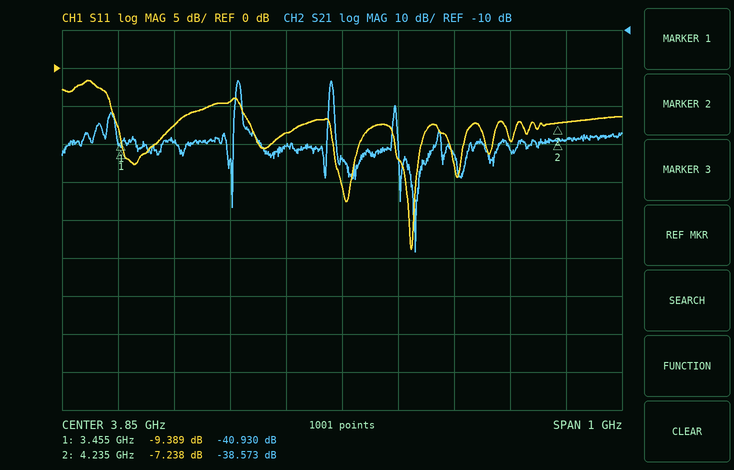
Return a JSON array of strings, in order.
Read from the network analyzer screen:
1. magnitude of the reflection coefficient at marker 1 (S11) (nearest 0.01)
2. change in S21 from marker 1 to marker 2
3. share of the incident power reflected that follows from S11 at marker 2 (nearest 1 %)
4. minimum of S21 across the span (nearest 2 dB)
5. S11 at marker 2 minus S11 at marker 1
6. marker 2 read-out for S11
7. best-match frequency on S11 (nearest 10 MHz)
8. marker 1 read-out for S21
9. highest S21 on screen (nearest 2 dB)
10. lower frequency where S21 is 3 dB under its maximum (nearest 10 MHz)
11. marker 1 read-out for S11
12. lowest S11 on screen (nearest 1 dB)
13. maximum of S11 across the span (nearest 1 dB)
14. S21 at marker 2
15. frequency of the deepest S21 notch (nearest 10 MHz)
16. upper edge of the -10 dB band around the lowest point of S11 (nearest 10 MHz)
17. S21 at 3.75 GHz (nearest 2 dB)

["0.34", "2.357 dB", "19 %", "-68 dB", "2.151 dB", "-7.238 dB", "3.97 GHz", "-40.930 dB", "-24 dB", "3.66 GHz", "-9.389 dB", "-24 dB", "-2 dB", "-38.573 dB", "3.98 GHz", "3.99 GHz", "-40 dB"]
